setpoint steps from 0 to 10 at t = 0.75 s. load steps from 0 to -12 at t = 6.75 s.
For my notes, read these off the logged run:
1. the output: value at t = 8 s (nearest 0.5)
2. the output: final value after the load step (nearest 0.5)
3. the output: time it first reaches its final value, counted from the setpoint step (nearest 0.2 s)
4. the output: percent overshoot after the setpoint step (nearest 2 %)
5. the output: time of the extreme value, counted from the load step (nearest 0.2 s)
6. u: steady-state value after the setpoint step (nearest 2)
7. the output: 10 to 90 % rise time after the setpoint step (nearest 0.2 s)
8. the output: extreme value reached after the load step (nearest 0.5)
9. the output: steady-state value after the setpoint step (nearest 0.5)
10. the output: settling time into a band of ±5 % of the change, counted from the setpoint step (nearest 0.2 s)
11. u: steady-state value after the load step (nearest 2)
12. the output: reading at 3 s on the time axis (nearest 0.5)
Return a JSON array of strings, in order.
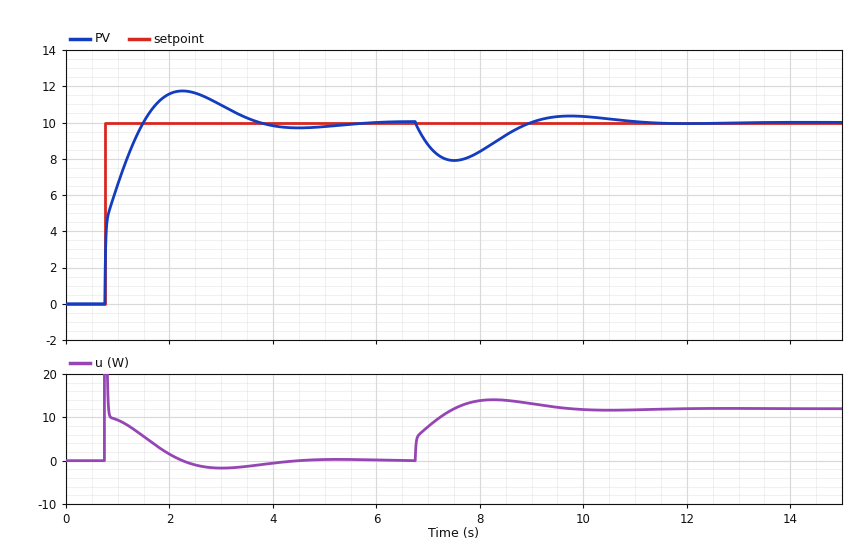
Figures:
["8.5", "10.0", "0.8 s", "18 %", "0.8 s", "0", "0.6 s", "8.0", "10.0", "2.6 s", "12", "11.0"]
